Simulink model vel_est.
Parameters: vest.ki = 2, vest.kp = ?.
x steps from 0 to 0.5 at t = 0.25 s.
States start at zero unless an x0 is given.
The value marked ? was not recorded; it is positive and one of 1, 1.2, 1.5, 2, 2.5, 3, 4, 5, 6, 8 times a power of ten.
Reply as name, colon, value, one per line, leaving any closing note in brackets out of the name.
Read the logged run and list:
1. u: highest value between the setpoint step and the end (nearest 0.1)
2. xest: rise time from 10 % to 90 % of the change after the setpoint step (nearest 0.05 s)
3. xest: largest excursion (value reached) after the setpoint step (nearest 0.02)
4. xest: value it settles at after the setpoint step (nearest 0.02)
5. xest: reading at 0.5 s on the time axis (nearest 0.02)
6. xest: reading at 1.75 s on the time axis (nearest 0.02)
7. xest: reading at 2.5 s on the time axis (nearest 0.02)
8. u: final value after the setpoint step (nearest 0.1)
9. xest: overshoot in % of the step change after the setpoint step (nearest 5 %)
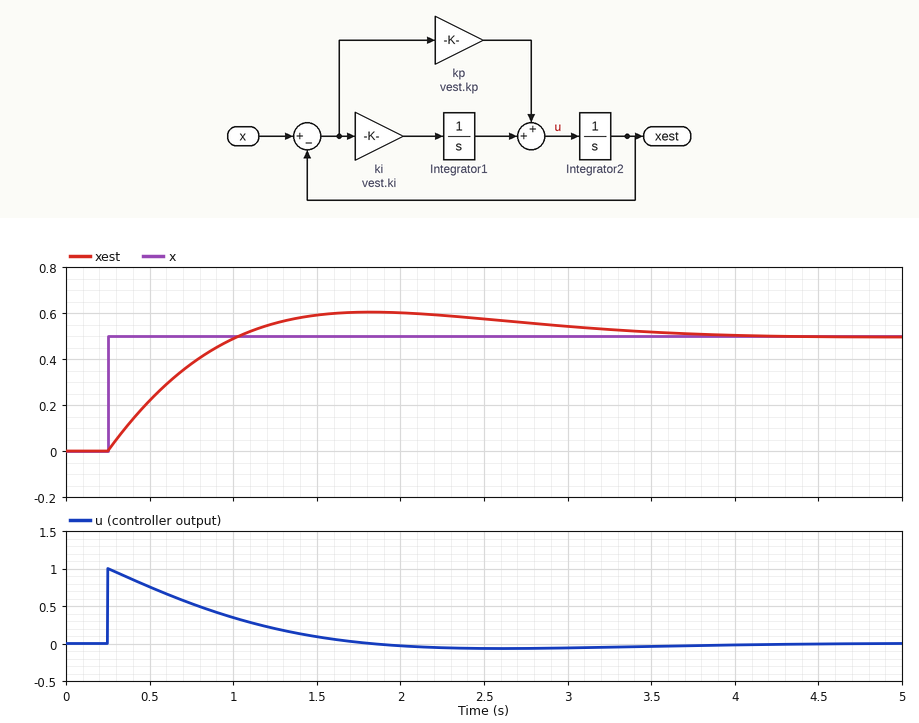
u: highest value between the setpoint step and the end: 1.0
xest: rise time from 10 % to 90 % of the change after the setpoint step: 0.60 s
xest: largest excursion (value reached) after the setpoint step: 0.60
xest: value it settles at after the setpoint step: 0.50
xest: reading at 0.5 s on the time axis: 0.22
xest: reading at 1.75 s on the time axis: 0.60
xest: reading at 2.5 s on the time axis: 0.58
u: final value after the setpoint step: 0.0
xest: overshoot in % of the step change after the setpoint step: 20 %
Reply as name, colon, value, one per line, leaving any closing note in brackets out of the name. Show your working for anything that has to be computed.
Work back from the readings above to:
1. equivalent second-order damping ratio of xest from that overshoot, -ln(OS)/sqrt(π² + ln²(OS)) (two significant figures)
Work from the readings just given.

equivalent second-order damping ratio of xest from that overshoot, -ln(OS)/sqrt(π² + ln²(OS)): ln(0.2) = -1.609; 1.609 / sqrt(9.870 + 2.590) = 0.46
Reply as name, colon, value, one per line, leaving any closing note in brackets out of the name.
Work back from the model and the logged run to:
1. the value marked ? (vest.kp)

the value marked ?: 2
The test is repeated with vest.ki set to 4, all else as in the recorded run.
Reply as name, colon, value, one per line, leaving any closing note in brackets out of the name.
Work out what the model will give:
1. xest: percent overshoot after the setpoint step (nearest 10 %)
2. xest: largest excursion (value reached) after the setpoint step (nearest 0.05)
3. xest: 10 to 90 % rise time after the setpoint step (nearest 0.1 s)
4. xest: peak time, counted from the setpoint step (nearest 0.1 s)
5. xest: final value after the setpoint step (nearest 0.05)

xest: percent overshoot after the setpoint step: 30 %
xest: largest excursion (value reached) after the setpoint step: 0.65
xest: 10 to 90 % rise time after the setpoint step: 0.5 s
xest: peak time, counted from the setpoint step: 1.2 s
xest: final value after the setpoint step: 0.50
